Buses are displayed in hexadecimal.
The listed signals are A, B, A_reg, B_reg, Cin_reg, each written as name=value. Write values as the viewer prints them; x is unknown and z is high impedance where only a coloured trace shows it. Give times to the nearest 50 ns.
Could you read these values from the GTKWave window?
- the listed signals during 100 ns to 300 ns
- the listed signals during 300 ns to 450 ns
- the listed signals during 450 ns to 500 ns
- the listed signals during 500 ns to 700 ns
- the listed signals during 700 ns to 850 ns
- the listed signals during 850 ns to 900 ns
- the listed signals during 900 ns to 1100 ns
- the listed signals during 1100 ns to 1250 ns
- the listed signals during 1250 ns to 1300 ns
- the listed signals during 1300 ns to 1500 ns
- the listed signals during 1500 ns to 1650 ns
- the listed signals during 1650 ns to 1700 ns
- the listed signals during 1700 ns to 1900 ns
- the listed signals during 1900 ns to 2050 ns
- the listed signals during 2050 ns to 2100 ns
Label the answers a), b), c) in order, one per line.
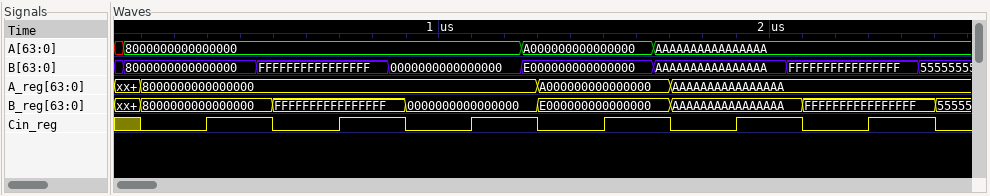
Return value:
a) A=8000000000000000, B=8000000000000000, A_reg=8000000000000000, B_reg=8000000000000000, Cin_reg=0
b) A=8000000000000000, B=8000000000000000, A_reg=8000000000000000, B_reg=8000000000000000, Cin_reg=1
c) A=8000000000000000, B=FFFFFFFFFFFFFFFF, A_reg=8000000000000000, B_reg=8000000000000000, Cin_reg=1
d) A=8000000000000000, B=FFFFFFFFFFFFFFFF, A_reg=8000000000000000, B_reg=FFFFFFFFFFFFFFFF, Cin_reg=0
e) A=8000000000000000, B=FFFFFFFFFFFFFFFF, A_reg=8000000000000000, B_reg=FFFFFFFFFFFFFFFF, Cin_reg=1
f) A=8000000000000000, B=0000000000000000, A_reg=8000000000000000, B_reg=FFFFFFFFFFFFFFFF, Cin_reg=1
g) A=8000000000000000, B=0000000000000000, A_reg=8000000000000000, B_reg=0000000000000000, Cin_reg=0
h) A=8000000000000000, B=0000000000000000, A_reg=8000000000000000, B_reg=0000000000000000, Cin_reg=1
i) A=A000000000000000, B=E000000000000000, A_reg=8000000000000000, B_reg=0000000000000000, Cin_reg=1
j) A=A000000000000000, B=E000000000000000, A_reg=A000000000000000, B_reg=E000000000000000, Cin_reg=0
k) A=A000000000000000, B=E000000000000000, A_reg=A000000000000000, B_reg=E000000000000000, Cin_reg=1
l) A=AAAAAAAAAAAAAAAA, B=AAAAAAAAAAAAAAAA, A_reg=A000000000000000, B_reg=E000000000000000, Cin_reg=1
m) A=AAAAAAAAAAAAAAAA, B=AAAAAAAAAAAAAAAA, A_reg=AAAAAAAAAAAAAAAA, B_reg=AAAAAAAAAAAAAAAA, Cin_reg=0
n) A=AAAAAAAAAAAAAAAA, B=AAAAAAAAAAAAAAAA, A_reg=AAAAAAAAAAAAAAAA, B_reg=AAAAAAAAAAAAAAAA, Cin_reg=1
o) A=AAAAAAAAAAAAAAAA, B=FFFFFFFFFFFFFFFF, A_reg=AAAAAAAAAAAAAAAA, B_reg=AAAAAAAAAAAAAAAA, Cin_reg=1
